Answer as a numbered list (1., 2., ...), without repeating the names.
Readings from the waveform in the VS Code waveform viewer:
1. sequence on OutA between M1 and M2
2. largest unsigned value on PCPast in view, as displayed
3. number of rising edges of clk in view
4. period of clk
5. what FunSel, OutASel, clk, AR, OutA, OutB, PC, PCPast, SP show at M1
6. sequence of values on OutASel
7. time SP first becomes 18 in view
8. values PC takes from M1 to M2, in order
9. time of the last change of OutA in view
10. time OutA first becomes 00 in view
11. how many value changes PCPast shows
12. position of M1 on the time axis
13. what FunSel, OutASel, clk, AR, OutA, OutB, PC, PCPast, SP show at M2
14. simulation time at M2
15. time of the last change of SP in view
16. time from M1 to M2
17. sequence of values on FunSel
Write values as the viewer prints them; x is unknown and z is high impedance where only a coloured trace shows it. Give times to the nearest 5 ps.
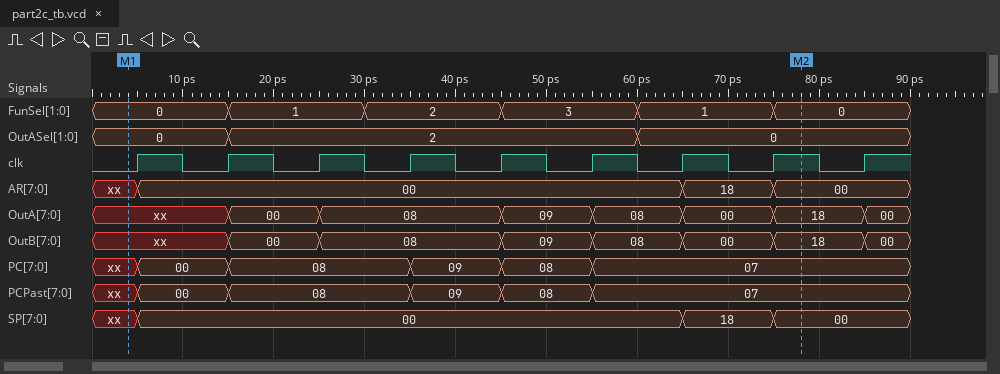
1. xx, 00, 08, 09, 08, 00, 18
2. 09
3. 9
4. 10 ps
5. FunSel=0, OutASel=0, clk=0, AR=xx, OutA=xx, OutB=xx, PC=xx, PCPast=xx, SP=xx
6. 0, 2, 0
7. 65 ps
8. xx, 00, 08, 09, 08, 07
9. 85 ps
10. 15 ps
11. 5
12. 5 ps
13. FunSel=0, OutASel=0, clk=1, AR=00, OutA=18, OutB=18, PC=07, PCPast=07, SP=00
14. 80 ps
15. 75 ps
16. 75 ps
17. 0, 1, 2, 3, 1, 0
